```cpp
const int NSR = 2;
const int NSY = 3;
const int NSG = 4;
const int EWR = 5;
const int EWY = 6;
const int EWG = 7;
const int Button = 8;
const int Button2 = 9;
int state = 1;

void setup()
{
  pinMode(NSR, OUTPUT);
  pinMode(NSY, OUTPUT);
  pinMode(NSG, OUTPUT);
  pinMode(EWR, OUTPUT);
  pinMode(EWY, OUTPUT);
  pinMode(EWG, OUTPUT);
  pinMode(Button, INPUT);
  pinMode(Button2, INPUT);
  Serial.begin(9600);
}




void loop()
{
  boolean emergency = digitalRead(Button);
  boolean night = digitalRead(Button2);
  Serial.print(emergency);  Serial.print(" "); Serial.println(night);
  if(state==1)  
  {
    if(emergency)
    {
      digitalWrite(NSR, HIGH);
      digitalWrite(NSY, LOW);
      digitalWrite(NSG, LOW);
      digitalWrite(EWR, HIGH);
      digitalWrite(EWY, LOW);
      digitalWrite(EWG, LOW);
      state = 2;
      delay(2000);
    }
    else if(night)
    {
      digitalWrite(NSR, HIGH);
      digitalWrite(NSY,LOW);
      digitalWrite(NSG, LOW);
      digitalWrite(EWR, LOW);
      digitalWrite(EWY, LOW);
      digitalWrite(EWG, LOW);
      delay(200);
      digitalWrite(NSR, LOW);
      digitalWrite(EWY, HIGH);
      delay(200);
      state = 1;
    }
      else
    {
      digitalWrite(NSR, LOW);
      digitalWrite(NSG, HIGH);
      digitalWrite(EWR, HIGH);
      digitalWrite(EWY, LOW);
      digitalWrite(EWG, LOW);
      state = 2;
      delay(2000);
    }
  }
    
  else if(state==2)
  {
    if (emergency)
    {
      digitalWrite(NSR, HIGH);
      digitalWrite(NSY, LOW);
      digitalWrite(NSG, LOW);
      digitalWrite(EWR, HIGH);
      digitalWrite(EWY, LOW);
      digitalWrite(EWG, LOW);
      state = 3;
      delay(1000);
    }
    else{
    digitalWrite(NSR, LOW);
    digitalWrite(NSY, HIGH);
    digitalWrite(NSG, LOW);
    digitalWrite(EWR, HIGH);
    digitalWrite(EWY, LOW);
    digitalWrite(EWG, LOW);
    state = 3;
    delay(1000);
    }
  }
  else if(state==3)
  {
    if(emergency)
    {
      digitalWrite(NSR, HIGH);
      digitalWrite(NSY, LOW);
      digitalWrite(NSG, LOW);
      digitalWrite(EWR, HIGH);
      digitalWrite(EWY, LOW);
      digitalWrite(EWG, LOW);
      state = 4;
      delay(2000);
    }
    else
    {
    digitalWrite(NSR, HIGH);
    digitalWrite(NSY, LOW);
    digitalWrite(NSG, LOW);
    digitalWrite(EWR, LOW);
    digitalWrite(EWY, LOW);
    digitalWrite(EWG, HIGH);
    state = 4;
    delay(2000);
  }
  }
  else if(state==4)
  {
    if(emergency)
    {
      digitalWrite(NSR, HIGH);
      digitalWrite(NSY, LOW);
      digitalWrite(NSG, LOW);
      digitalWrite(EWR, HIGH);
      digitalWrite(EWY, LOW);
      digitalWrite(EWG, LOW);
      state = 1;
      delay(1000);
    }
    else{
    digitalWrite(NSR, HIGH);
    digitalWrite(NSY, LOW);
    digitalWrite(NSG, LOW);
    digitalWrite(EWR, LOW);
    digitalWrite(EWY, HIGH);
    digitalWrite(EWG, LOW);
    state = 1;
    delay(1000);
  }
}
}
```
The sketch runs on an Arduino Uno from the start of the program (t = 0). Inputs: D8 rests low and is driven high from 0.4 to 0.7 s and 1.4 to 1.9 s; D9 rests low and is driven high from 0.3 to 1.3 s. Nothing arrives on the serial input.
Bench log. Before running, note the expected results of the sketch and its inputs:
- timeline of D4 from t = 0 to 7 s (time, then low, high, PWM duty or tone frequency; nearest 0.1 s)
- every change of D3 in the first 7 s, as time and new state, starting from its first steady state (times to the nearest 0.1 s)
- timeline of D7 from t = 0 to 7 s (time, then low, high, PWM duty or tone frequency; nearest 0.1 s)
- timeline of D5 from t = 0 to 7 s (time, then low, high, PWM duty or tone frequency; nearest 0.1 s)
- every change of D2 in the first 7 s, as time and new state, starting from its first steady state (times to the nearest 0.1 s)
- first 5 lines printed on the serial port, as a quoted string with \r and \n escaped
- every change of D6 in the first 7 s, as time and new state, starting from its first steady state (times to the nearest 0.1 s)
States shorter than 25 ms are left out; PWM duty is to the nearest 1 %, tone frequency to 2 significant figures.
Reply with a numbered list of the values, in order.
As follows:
1. 0 s high; 2 s low; 6 s high
2. 0 s low; 2 s high; 3 s low
3. 0 s low; 3 s high; 5 s low
4. 0 s high; 3 s low; 6 s high
5. 0 s low; 3 s high; 6 s low
6. "0 0\r\n0 0\r\n0 0\r\n0 0\r\n0 0\r\n"
7. 0 s low; 5 s high; 6 s low
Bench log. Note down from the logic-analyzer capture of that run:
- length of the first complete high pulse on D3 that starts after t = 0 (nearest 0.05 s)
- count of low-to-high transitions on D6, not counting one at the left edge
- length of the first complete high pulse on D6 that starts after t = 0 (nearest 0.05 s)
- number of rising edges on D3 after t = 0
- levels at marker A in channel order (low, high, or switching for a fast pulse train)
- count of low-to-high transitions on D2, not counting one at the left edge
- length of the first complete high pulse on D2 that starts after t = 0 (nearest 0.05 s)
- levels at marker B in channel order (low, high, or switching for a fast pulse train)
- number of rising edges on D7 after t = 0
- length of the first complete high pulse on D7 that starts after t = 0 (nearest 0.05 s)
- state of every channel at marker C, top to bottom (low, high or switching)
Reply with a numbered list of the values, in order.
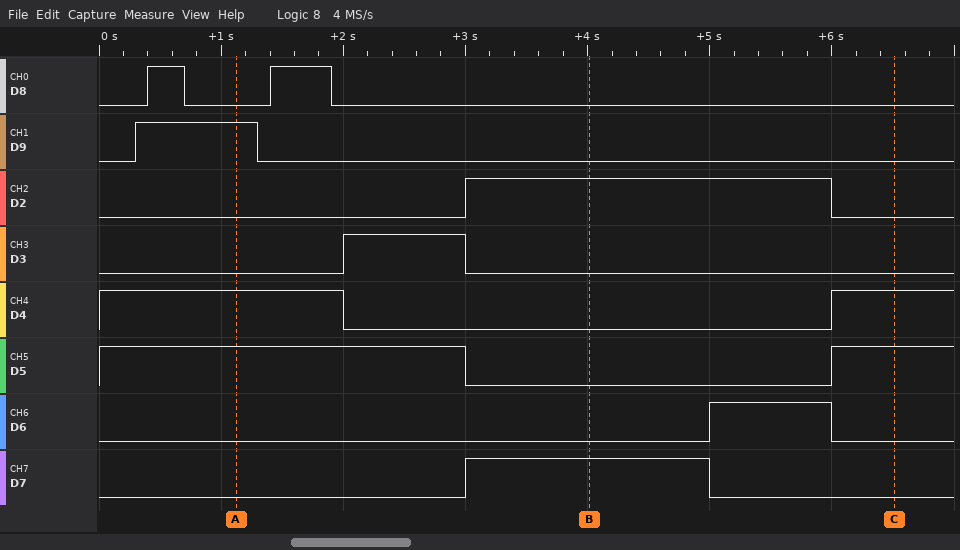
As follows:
1. 1.00 s
2. 1
3. 1.00 s
4. 1
5. D8 low, D9 high, D2 low, D3 low, D4 high, D5 high, D6 low, D7 low
6. 1
7. 3.00 s
8. D8 low, D9 low, D2 high, D3 low, D4 low, D5 low, D6 low, D7 high
9. 1
10. 2.00 s
11. D8 low, D9 low, D2 low, D3 low, D4 high, D5 high, D6 low, D7 low
